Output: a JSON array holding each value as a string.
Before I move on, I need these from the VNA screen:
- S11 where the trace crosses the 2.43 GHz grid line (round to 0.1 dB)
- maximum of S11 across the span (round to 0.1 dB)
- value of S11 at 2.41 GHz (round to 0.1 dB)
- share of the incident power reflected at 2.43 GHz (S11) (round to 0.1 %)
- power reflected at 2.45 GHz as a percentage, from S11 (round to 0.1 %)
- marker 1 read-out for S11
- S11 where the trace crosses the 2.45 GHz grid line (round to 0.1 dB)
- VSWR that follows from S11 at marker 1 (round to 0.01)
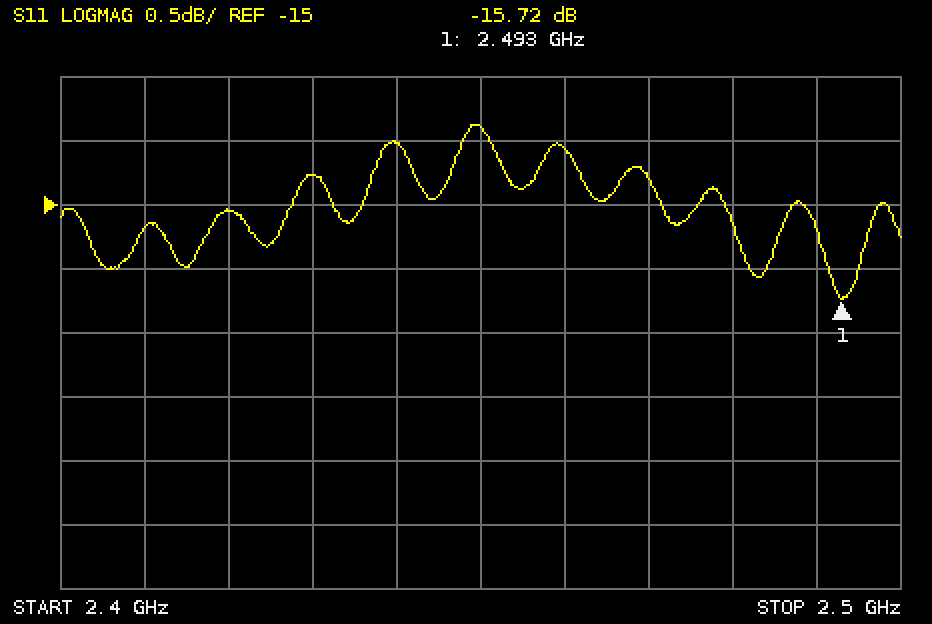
["-14.8 dB", "-14.4 dB", "-15.2 dB", "3.3 %", "3.6 %", "-15.72 dB", "-14.4 dB", "1.39"]
